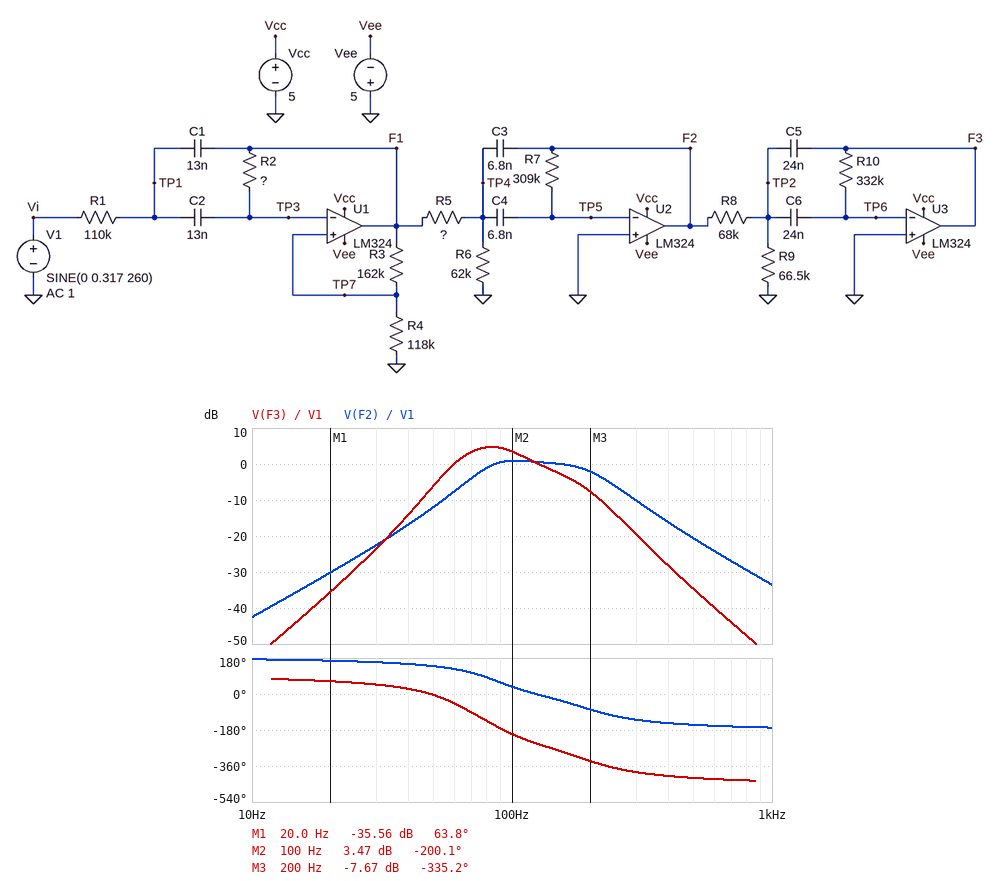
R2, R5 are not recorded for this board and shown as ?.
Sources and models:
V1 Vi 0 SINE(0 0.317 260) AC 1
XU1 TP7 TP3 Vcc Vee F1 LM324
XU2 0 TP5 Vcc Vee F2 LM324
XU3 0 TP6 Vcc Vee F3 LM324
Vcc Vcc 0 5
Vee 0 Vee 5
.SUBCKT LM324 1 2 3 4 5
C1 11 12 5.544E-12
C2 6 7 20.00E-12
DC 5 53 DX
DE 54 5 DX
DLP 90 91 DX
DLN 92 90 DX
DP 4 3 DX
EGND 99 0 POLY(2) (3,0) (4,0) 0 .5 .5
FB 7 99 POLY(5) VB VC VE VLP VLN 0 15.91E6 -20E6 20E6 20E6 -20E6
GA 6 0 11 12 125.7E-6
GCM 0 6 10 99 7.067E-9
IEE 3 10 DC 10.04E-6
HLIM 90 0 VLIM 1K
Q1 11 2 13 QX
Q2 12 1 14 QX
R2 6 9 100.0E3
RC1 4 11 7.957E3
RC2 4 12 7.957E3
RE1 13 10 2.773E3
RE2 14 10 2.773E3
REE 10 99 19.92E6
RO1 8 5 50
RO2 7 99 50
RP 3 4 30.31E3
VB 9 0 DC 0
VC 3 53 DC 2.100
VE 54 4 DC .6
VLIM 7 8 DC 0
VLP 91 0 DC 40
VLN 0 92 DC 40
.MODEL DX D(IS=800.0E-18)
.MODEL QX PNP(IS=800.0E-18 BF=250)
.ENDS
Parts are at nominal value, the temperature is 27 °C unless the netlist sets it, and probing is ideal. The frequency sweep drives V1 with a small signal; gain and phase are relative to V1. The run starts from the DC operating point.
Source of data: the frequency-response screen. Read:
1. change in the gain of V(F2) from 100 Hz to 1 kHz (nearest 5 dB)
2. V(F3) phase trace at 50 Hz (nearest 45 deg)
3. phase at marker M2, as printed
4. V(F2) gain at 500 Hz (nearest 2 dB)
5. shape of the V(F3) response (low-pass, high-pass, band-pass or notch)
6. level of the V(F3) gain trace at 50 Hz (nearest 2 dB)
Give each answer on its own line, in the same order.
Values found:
-35 dB
0 deg
-200.1 deg
-20 dB
band-pass
-6 dB
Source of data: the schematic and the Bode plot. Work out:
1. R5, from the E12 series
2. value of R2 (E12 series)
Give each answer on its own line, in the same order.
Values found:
220 kΩ
180 kΩ
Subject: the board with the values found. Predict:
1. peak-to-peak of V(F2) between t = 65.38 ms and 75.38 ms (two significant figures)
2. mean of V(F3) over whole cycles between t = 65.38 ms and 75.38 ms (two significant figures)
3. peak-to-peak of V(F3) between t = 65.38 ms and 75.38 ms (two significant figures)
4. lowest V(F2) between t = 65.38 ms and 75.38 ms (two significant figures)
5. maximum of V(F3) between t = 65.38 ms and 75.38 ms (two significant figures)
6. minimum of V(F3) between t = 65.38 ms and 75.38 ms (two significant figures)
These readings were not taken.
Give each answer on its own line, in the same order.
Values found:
280 mV
-6.6 mV
110 mV
-150 mV
49 mV
-62 mV
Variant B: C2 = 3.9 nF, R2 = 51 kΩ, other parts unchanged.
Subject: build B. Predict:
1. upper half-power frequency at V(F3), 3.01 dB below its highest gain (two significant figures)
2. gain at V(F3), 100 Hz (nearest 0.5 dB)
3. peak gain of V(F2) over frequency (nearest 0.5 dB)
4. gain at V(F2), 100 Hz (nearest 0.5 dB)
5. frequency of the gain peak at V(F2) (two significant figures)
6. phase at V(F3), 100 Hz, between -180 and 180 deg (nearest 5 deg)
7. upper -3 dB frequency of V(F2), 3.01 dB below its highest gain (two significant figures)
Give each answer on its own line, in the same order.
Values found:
230 Hz
-23.0 dB
-17.5 dB
-25.5 dB
200 Hz
-135 deg
290 Hz
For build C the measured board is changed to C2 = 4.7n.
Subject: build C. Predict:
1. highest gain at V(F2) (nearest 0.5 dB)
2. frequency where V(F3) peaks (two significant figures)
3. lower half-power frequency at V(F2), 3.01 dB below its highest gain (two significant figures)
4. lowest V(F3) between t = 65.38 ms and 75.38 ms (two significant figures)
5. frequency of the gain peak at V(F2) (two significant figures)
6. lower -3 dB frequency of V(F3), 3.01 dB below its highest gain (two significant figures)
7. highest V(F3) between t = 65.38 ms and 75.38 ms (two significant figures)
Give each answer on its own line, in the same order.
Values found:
-3.0 dB
140 Hz
130 Hz
-59 mV
180 Hz
71 Hz
46 mV
